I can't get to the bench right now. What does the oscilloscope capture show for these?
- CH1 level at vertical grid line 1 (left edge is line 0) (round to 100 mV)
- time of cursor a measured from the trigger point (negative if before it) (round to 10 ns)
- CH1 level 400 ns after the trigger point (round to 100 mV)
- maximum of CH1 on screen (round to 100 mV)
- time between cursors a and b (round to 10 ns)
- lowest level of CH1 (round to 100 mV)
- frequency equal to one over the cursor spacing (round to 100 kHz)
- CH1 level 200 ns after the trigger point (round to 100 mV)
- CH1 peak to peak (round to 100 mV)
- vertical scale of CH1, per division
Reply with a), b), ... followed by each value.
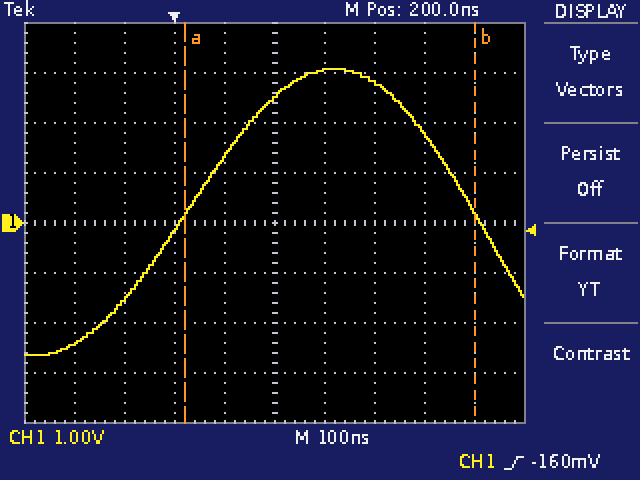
a) -2.4 V
b) +20 ns
c) 2.8 V
d) 3.1 V
e) 580 ns
f) -2.6 V
g) 1.7 MHz
h) 2.5 V
i) 5.7 V
j) 1 V
